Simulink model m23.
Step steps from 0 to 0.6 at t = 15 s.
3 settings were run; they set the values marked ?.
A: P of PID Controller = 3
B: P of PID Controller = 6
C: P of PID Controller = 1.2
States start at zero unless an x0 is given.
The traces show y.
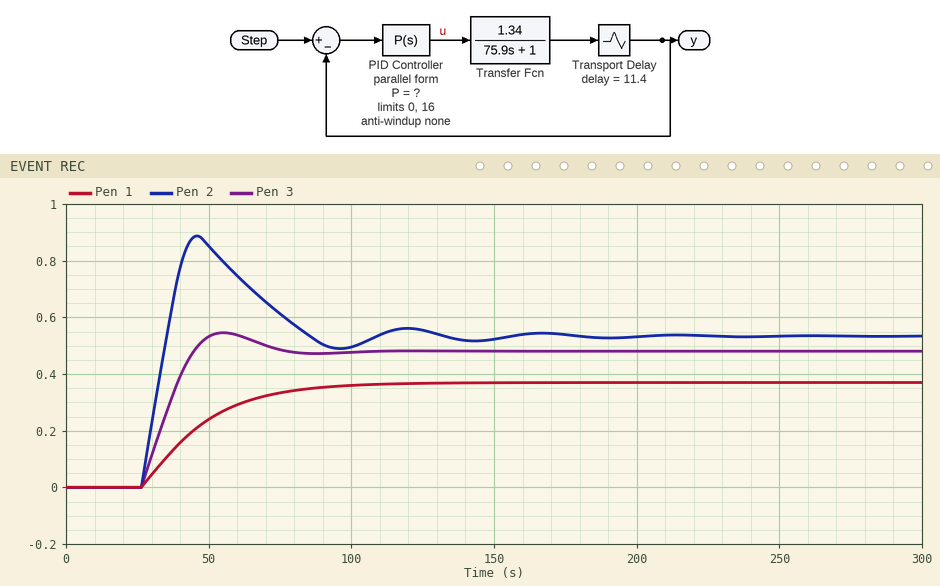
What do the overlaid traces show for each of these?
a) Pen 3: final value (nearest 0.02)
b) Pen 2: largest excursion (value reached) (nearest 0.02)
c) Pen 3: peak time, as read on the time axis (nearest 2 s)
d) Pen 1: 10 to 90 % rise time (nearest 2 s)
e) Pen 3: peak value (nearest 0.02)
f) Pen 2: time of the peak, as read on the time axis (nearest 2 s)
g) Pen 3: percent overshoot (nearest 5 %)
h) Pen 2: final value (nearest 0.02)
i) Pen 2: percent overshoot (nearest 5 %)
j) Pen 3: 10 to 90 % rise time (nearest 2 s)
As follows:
0.48
0.88
56 s
46 s
0.54
46 s
15 %
0.54
65 %
14 s
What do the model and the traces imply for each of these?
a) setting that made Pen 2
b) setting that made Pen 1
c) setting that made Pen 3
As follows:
B
C
A
